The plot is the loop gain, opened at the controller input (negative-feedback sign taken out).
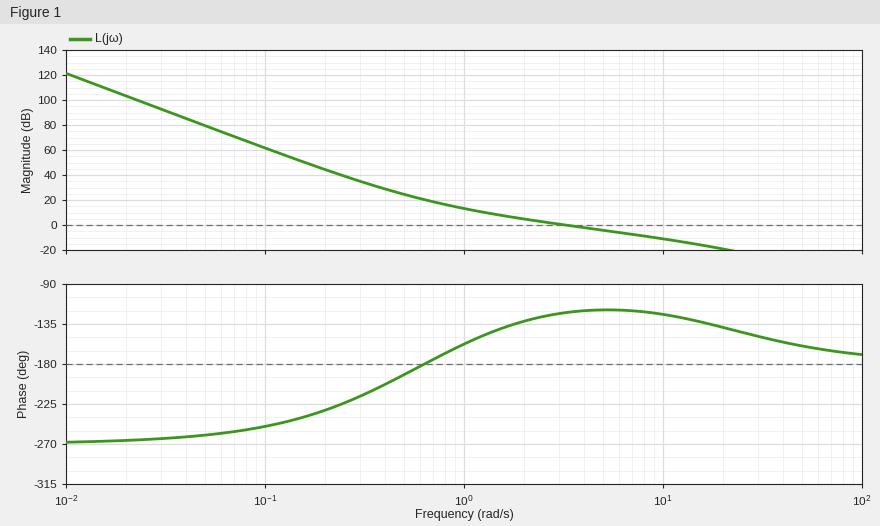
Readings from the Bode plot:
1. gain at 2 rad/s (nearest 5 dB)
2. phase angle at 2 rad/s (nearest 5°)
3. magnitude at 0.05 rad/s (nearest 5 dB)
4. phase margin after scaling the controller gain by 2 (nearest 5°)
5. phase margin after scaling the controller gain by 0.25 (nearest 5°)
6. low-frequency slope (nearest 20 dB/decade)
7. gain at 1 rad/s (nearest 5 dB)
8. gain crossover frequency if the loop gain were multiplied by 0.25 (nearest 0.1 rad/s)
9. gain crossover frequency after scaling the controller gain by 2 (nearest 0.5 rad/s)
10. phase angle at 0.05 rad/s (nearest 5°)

5 dB
-130°
80 dB
60°
25°
-60 dB/decade
15 dB
1.1 rad/s
6.0 rad/s
-260°
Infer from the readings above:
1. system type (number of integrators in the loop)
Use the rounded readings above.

3
